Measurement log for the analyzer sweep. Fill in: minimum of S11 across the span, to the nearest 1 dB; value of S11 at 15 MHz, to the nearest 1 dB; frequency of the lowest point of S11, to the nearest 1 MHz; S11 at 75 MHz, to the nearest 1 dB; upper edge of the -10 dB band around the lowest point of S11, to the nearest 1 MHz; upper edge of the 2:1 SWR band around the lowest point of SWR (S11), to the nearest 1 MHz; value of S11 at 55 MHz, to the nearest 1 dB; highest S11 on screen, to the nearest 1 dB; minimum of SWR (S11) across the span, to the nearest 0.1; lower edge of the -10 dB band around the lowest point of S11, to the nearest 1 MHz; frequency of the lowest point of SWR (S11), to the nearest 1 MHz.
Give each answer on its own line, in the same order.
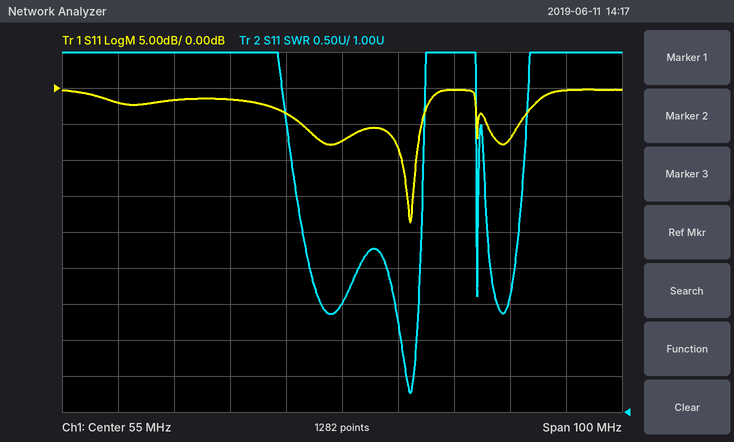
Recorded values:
-19 dB
-2 dB
67 MHz
0 dB
68 MHz
68 MHz
-7 dB
0 dB
1.3
66 MHz
67 MHz
